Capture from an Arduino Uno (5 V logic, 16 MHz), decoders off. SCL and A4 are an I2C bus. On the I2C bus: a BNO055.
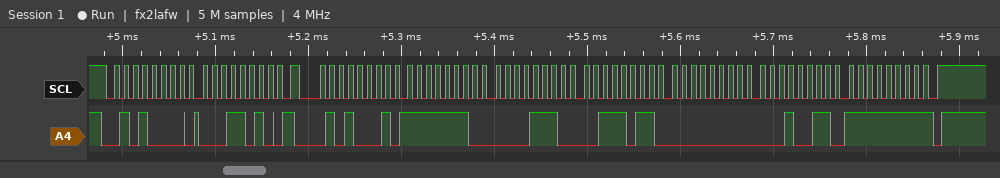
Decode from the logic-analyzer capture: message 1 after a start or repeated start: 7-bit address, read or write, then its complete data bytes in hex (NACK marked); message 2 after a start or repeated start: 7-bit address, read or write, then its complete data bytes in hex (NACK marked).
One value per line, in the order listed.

0x28 write: 1A
0x28 read: FE 0E 3B 00 13 FF NACK
